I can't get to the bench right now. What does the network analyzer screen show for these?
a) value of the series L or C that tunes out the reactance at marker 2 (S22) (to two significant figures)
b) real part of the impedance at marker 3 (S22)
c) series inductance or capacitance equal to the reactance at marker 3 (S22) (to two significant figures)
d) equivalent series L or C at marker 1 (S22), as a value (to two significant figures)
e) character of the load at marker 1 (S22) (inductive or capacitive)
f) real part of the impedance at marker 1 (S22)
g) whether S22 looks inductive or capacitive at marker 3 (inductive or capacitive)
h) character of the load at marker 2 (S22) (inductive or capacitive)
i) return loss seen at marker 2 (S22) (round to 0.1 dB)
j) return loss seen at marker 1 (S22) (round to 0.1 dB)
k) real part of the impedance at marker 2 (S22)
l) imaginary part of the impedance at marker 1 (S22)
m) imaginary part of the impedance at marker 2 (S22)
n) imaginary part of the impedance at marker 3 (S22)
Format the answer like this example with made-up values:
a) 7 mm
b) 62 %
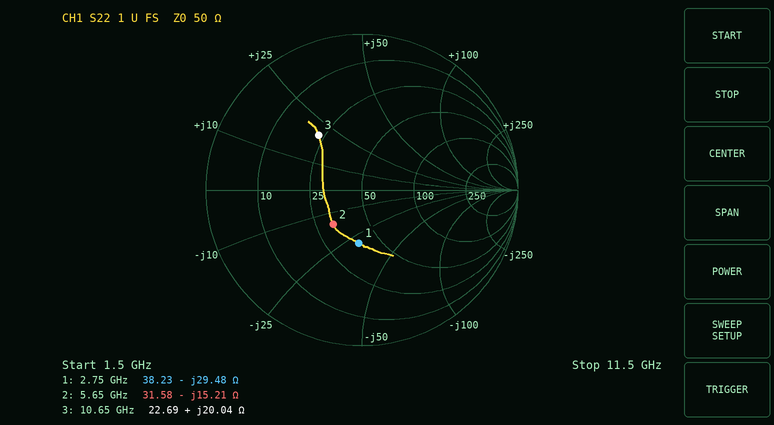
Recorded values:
a) 430 pH
b) 22.69 Ω
c) 300 pH
d) 2.0 pF
e) capacitive
f) 38.23 Ω
g) inductive
h) capacitive
i) 10.8 dB
j) 9.3 dB
k) 31.58 Ω
l) -29.48 Ω
m) -15.21 Ω
n) +20.04 Ω
